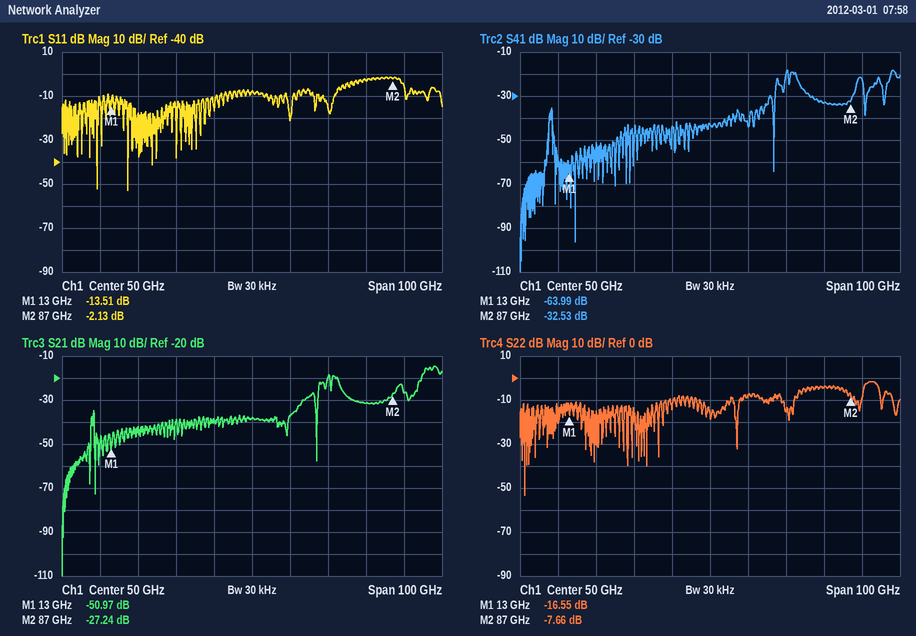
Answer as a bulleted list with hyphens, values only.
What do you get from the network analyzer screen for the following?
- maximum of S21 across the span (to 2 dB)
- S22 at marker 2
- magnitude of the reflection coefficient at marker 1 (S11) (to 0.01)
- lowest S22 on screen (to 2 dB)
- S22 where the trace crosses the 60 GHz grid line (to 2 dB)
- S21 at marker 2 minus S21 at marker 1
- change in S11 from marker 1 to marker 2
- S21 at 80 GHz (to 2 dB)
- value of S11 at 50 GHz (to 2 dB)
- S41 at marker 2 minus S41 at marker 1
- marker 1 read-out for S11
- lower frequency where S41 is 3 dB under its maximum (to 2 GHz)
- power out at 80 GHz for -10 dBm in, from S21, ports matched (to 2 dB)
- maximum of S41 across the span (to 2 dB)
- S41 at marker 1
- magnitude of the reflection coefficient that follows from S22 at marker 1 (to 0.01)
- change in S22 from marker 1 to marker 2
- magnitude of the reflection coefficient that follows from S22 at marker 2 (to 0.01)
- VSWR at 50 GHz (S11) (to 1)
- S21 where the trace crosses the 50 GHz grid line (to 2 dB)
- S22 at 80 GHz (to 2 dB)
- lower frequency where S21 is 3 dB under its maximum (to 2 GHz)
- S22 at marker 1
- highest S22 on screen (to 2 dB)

- -14 dB
- -7.66 dB
- 0.21
- -54 dB
- -8 dB
- 23.73 dB
- 11.38 dB
- -32 dB
- -8 dB
- 31.46 dB
- -13.51 dB
- 70 GHz
- -42 dBm
- -18 dB
- -63.99 dB
- 0.15
- 8.89 dB
- 0.41
- 2
- -38 dB
- -4 dB
- 96 GHz
- -16.55 dB
- -2 dB
